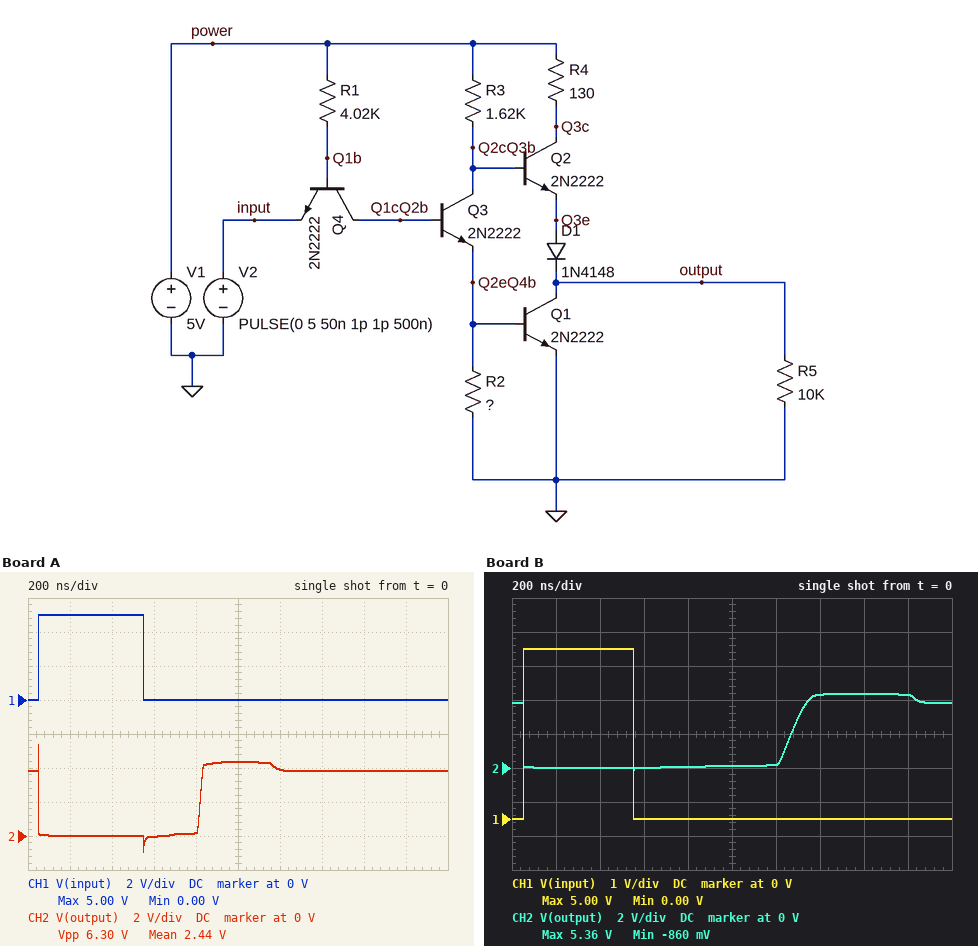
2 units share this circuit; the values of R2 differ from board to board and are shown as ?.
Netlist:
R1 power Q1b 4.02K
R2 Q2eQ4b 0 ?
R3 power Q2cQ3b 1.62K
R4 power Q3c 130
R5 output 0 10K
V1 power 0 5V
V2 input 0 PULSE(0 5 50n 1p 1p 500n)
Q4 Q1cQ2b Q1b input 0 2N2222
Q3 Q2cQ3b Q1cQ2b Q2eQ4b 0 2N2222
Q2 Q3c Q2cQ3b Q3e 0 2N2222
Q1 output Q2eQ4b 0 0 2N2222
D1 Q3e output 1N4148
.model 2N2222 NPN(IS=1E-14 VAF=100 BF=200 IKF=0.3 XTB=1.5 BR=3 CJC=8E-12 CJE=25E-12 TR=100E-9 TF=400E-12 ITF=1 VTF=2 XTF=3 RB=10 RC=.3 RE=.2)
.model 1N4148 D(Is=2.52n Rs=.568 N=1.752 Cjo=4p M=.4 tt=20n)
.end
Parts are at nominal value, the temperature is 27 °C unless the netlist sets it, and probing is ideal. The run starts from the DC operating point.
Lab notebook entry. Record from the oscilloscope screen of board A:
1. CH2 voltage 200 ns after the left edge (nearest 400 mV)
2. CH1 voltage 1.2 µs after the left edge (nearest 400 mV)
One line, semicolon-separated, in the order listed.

0 V; 0 V
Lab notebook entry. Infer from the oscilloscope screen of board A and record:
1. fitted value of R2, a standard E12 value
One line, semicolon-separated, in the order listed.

470 Ω
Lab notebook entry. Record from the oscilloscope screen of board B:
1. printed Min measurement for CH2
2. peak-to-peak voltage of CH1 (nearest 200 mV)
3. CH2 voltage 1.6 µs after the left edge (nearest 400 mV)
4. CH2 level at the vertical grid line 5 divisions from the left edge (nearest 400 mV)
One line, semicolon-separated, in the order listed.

-860 mV; 5.0 V; 4.4 V; 0 V
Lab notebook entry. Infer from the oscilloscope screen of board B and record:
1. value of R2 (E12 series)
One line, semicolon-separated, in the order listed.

3.3 kΩ
